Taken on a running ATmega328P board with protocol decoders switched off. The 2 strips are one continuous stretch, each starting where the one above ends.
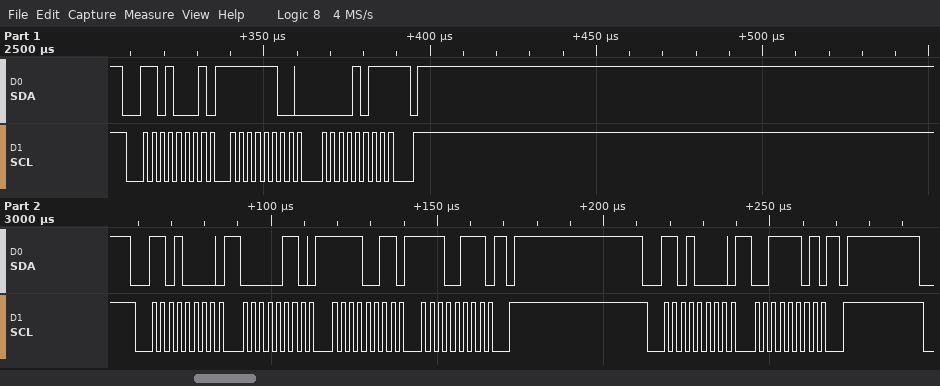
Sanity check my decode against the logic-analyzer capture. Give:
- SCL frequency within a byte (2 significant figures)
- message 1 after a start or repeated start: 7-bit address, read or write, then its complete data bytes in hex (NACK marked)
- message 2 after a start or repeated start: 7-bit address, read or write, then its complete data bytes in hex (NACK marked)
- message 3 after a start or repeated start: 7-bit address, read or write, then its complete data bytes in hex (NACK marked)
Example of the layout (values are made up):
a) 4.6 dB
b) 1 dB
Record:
a) 400 kHz
b) 0x68 read: FC 0B NACK
c) 0x68 write: 06 F3 E7
d) 0x68 write: 3D
